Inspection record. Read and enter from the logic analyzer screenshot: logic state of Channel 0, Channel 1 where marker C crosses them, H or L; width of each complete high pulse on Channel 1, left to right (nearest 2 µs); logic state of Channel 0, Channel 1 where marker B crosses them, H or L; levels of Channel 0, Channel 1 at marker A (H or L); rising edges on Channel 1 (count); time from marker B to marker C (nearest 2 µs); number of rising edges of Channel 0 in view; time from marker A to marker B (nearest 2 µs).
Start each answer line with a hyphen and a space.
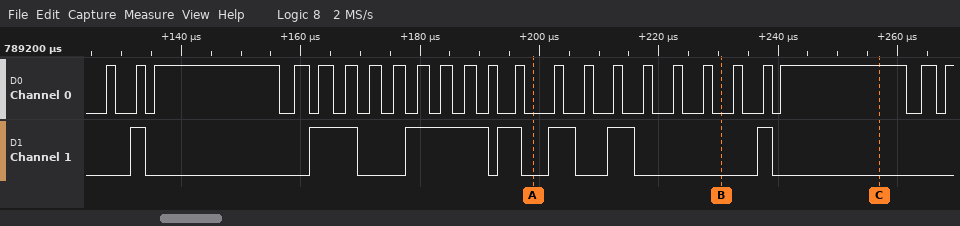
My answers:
- Channel 0=H, Channel 1=L
- 2 µs, 8 µs, 14 µs, 4 µs, 4 µs, 4 µs, 2 µs
- Channel 0=L, Channel 1=L
- Channel 0=L, Channel 1=L
- 7
- 26 µs
- 24
- 32 µs
